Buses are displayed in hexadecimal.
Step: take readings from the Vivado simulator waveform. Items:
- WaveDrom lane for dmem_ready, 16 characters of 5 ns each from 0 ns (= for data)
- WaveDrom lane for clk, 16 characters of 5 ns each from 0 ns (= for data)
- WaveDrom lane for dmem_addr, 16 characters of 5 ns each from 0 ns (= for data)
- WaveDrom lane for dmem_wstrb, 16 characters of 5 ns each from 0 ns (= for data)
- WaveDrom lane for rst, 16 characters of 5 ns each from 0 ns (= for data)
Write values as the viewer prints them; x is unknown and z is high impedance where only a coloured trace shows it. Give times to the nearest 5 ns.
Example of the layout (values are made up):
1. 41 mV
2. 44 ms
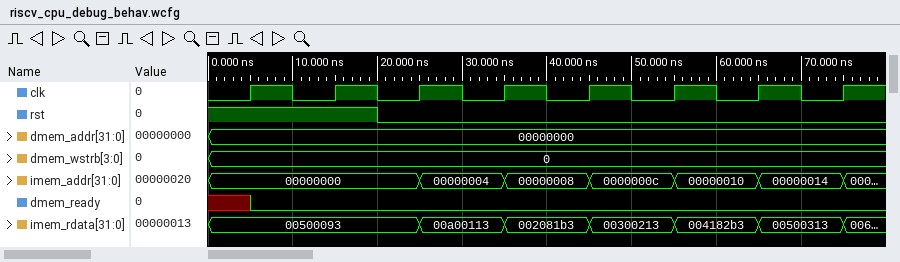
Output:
1. {name: 'dmem_ready', wave: 'x0..............'}
2. {name: 'clk', wave: '0101010101010101'}
3. {name: 'dmem_addr', wave: '=...............', data: '00000000'}
4. {name: 'dmem_wstrb', wave: '=...............', data: '0'}
5. {name: 'rst', wave: '1...0...........'}
